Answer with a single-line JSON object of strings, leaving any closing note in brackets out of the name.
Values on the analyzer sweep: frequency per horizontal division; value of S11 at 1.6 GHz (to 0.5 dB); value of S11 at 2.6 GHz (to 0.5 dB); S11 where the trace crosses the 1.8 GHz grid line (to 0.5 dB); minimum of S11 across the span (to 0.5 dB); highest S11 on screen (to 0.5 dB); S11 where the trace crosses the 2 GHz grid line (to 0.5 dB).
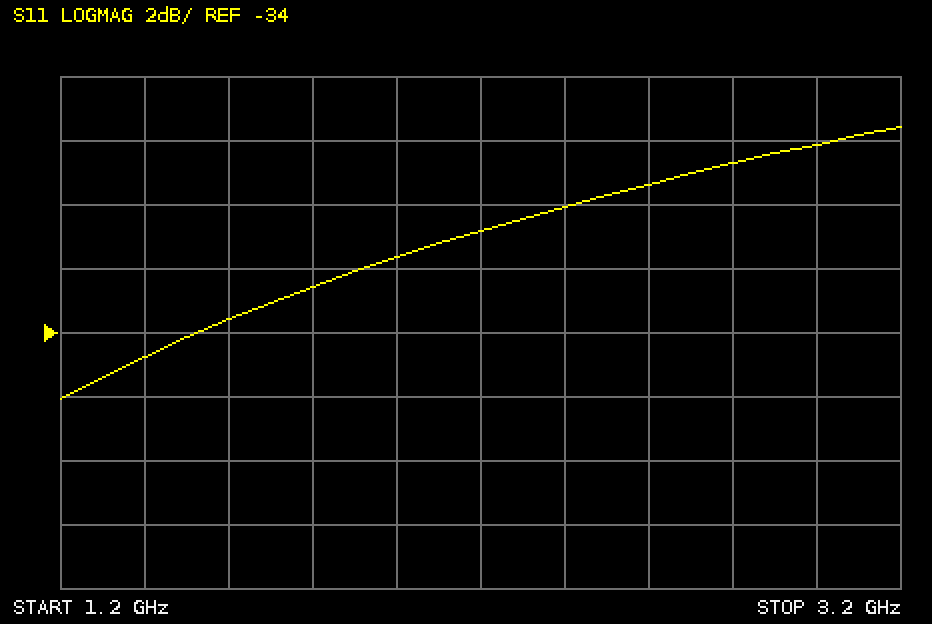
{"frequency per horizontal division": "200 MHz", "value of S11 at 1.6 GHz": "-33.5 dB", "value of S11 at 2.6 GHz": "-29.5 dB", "S11 where the trace crosses the 1.8 GHz grid line": "-32.5 dB", "minimum of S11 across the span": "-36.0 dB", "highest S11 on screen": "-27.5 dB", "S11 where the trace crosses the 2 GHz grid line": "-31.5 dB"}
